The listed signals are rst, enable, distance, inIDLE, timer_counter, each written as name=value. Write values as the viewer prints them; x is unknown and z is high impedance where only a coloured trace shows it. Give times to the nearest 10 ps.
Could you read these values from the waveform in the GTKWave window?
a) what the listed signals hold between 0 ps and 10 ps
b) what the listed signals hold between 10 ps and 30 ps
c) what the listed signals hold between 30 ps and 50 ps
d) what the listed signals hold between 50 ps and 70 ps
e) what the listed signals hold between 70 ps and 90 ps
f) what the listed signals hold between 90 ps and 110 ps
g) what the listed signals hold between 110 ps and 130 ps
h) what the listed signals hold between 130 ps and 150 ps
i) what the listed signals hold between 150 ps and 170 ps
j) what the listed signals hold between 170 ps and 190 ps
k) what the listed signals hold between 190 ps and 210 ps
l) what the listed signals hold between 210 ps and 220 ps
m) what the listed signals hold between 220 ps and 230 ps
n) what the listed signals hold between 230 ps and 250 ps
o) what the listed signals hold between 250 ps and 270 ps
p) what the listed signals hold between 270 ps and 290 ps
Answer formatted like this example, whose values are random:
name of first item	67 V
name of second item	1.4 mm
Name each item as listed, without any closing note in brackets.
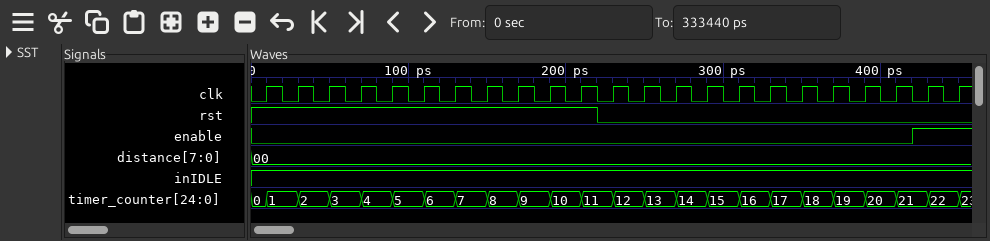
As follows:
what the listed signals hold between 0 ps and 10 ps	rst=1, enable=0, distance=00, inIDLE=1, timer_counter=0
what the listed signals hold between 10 ps and 30 ps	rst=1, enable=0, distance=00, inIDLE=1, timer_counter=1
what the listed signals hold between 30 ps and 50 ps	rst=1, enable=0, distance=00, inIDLE=1, timer_counter=2
what the listed signals hold between 50 ps and 70 ps	rst=1, enable=0, distance=00, inIDLE=1, timer_counter=3
what the listed signals hold between 70 ps and 90 ps	rst=1, enable=0, distance=00, inIDLE=1, timer_counter=4
what the listed signals hold between 90 ps and 110 ps	rst=1, enable=0, distance=00, inIDLE=1, timer_counter=5
what the listed signals hold between 110 ps and 130 ps	rst=1, enable=0, distance=00, inIDLE=1, timer_counter=6
what the listed signals hold between 130 ps and 150 ps	rst=1, enable=0, distance=00, inIDLE=1, timer_counter=7
what the listed signals hold between 150 ps and 170 ps	rst=1, enable=0, distance=00, inIDLE=1, timer_counter=8
what the listed signals hold between 170 ps and 190 ps	rst=1, enable=0, distance=00, inIDLE=1, timer_counter=9
what the listed signals hold between 190 ps and 210 ps	rst=1, enable=0, distance=00, inIDLE=1, timer_counter=10
what the listed signals hold between 210 ps and 220 ps	rst=1, enable=0, distance=00, inIDLE=1, timer_counter=11
what the listed signals hold between 220 ps and 230 ps	rst=0, enable=0, distance=00, inIDLE=1, timer_counter=11
what the listed signals hold between 230 ps and 250 ps	rst=0, enable=0, distance=00, inIDLE=1, timer_counter=12
what the listed signals hold between 250 ps and 270 ps	rst=0, enable=0, distance=00, inIDLE=1, timer_counter=13
what the listed signals hold between 270 ps and 290 ps	rst=0, enable=0, distance=00, inIDLE=1, timer_counter=14
